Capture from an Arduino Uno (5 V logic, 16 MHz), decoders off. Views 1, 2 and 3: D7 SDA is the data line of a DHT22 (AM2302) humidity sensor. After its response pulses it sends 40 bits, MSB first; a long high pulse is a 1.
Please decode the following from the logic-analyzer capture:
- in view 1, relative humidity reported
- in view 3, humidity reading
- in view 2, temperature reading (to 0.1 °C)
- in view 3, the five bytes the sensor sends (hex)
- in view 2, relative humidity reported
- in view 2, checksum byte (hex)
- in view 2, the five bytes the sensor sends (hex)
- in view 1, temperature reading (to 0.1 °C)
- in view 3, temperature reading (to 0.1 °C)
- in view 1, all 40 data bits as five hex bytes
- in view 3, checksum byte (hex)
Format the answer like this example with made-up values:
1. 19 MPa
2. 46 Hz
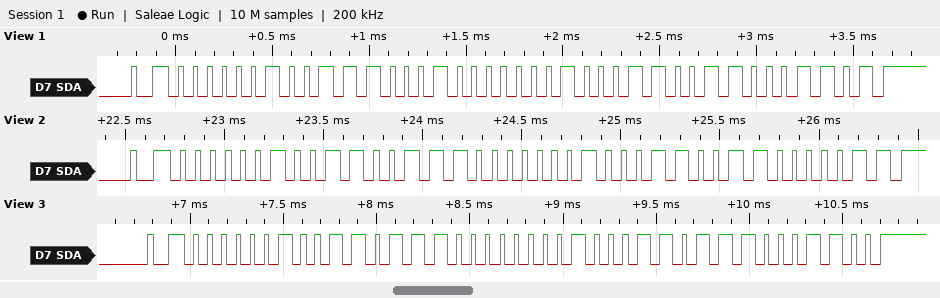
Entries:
1. 62.5 %
2. 62.2 %
3. 28.1 °C
4. 02 6E 01 1B 8C
5. 61.5 %
6. 0x83
7. 02 67 01 19 83
8. 28.1 °C
9. 28.3 °C
10. 02 71 01 19 8D
11. 0x8C
